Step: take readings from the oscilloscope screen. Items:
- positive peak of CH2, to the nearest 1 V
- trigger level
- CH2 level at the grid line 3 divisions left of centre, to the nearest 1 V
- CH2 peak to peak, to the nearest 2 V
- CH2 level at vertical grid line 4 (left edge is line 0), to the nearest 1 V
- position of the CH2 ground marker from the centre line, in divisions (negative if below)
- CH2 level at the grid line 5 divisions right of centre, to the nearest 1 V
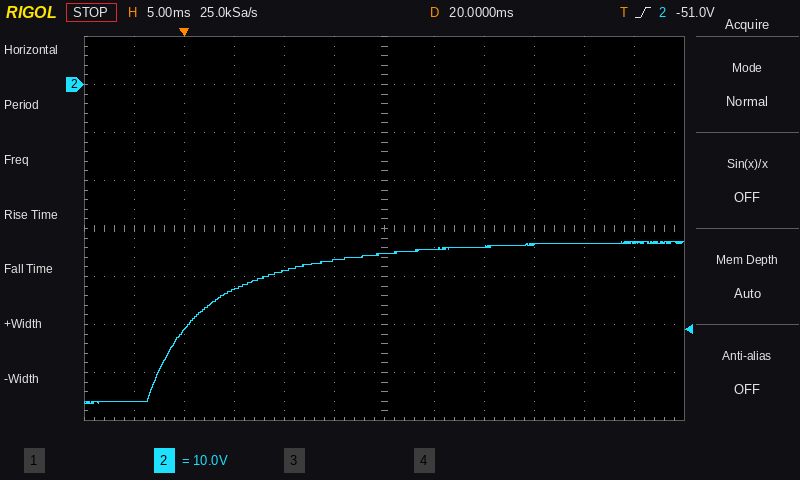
-33 V
-51.0 V
-43 V
34 V
-39 V
+3.0 div
-33 V
